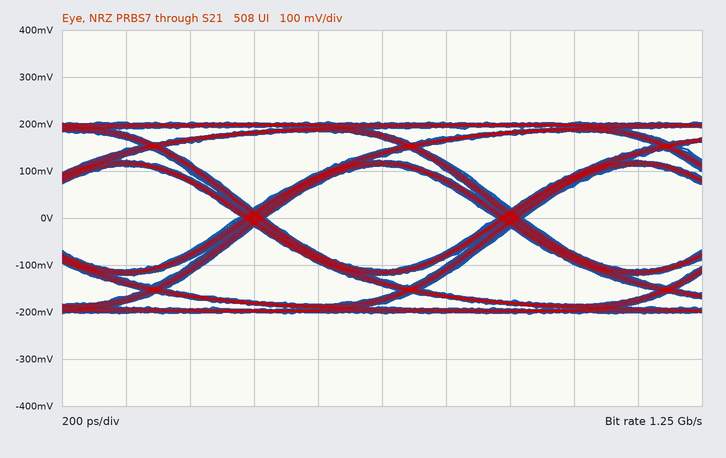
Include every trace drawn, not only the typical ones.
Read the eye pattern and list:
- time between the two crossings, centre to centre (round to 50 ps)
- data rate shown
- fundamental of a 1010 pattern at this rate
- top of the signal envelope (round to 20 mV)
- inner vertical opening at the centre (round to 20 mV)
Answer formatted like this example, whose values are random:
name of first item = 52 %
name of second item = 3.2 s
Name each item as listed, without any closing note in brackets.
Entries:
time between the two crossings, centre to centre = 800 ps
data rate shown = 1.25 Gb/s
fundamental of a 1010 pattern at this rate = 625 MHz
top of the signal envelope = 200 mV
inner vertical opening at the centre = 220 mV
